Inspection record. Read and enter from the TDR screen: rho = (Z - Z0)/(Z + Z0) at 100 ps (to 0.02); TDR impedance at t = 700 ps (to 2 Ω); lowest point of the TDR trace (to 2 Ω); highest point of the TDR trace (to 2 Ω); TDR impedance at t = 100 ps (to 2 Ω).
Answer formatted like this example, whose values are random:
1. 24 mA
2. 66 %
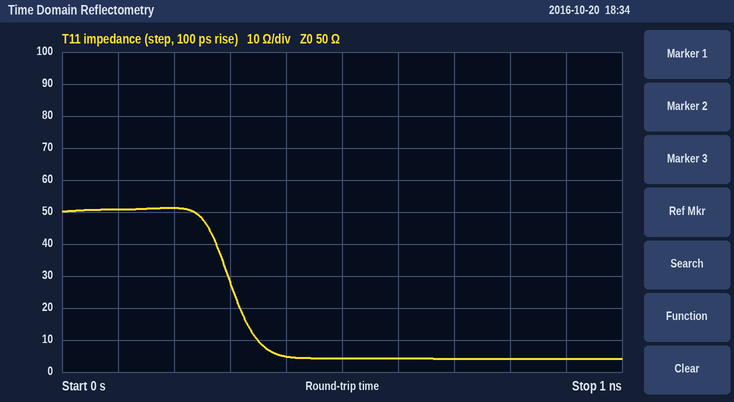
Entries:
1. 0.00
2. 4 Ω
3. 4 Ω
4. 52 Ω
5. 50 Ω
